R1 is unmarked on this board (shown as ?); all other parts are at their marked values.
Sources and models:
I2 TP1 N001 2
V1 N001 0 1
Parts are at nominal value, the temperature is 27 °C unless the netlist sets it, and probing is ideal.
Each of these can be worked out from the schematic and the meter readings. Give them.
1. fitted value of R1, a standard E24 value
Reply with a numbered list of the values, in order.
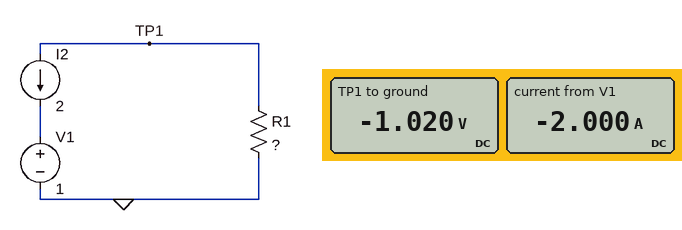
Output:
1. 0.51 Ω
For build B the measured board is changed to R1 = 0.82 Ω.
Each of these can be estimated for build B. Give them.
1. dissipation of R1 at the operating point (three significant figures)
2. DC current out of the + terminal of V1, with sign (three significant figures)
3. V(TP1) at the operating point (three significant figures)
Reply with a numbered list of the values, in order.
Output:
1. 3.28 W
2. -2.00 A
3. -1.64 V
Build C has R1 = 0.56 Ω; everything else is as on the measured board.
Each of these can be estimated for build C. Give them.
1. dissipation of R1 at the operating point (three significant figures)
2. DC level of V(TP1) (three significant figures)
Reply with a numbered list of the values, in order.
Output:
1. 2.24 W
2. -1.12 V
